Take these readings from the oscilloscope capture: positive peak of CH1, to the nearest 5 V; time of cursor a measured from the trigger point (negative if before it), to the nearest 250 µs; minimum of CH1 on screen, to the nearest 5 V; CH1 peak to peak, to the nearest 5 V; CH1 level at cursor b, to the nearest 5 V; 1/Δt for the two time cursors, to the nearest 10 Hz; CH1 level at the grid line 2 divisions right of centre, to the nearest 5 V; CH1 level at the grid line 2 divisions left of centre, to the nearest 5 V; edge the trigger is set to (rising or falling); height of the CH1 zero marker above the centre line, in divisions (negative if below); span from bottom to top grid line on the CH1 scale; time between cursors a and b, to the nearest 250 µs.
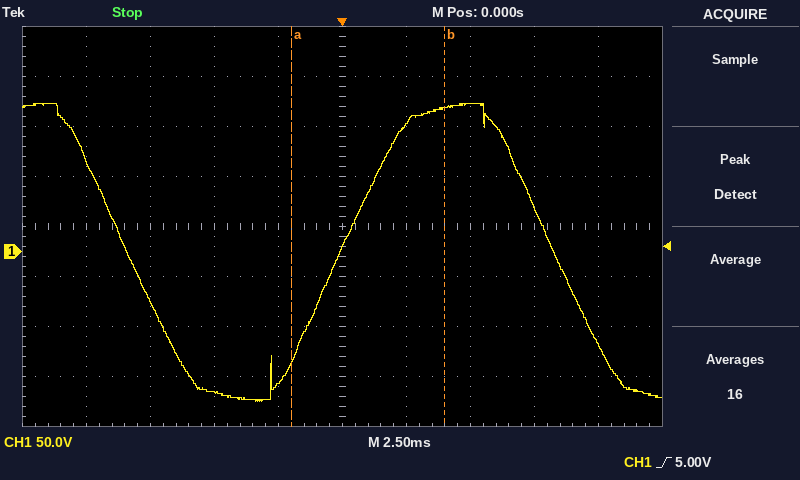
150 V
-2.00 ms
-150 V
300 V
145 V
170 Hz
150 V
-140 V
rising
-0.5 div
400 V
6.00 ms
